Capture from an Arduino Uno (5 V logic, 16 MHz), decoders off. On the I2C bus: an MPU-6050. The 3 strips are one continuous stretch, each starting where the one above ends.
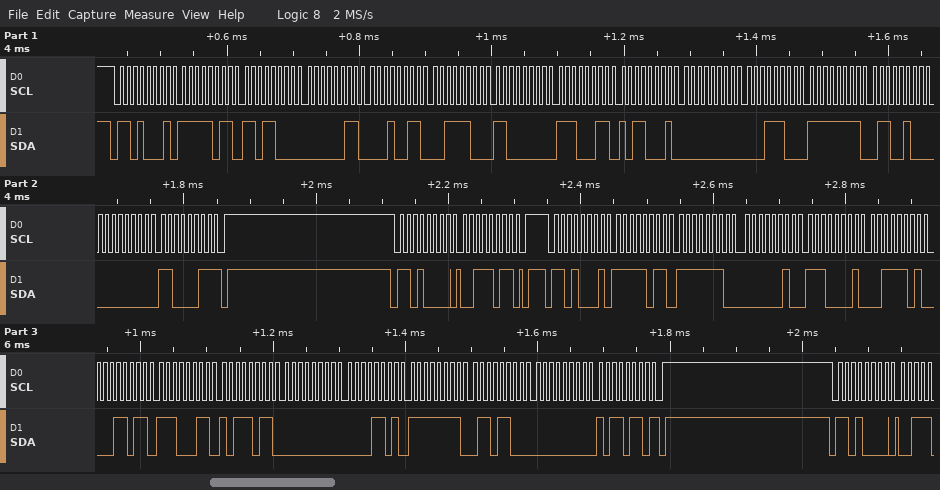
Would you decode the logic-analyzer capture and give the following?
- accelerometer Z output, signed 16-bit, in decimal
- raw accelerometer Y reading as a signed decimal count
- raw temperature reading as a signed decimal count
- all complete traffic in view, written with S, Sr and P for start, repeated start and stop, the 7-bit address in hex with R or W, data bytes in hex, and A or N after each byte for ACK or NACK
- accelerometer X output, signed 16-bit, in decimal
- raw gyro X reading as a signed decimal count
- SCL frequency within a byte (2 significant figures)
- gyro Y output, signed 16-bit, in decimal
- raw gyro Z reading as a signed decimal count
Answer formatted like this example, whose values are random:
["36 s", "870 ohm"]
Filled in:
["15643", "737", "-7237", "S 68R A FB A D8 A 03 A 13 A 3C A C0 A E3 A B1 A 00 A 1C A FF A 64 A 00 A C3 N P S 68W A 3B A P S 68R A FB A FE A 02 A E1 A 3D A 1B A E3 A BB A 00 A 0D A FF A 6C A 00 A B6 N P S 68W A", "-1026", "13", "100 kHz", "-148", "182"]
